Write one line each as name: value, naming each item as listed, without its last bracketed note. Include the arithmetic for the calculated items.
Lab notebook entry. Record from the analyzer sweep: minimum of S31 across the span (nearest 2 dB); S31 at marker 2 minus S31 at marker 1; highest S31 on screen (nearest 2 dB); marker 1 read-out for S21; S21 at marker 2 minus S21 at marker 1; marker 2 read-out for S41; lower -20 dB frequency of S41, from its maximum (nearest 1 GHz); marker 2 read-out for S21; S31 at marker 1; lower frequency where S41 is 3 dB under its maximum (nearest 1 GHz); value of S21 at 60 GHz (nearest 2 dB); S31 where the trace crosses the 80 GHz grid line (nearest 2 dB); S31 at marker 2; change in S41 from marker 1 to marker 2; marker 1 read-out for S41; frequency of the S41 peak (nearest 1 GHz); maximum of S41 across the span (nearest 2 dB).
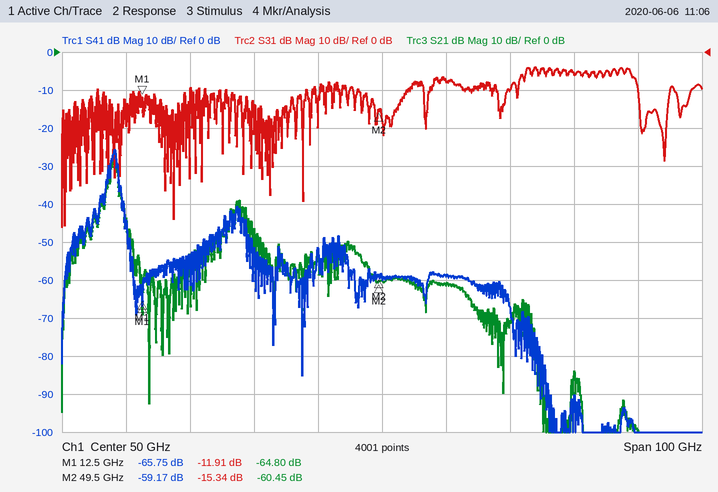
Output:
minimum of S31 across the span: -46 dB
S31 at marker 2 minus S31 at marker 1: -15.34 − (-11.91) = -3.43 dB
highest S31 on screen: -4 dB
marker 1 read-out for S21: -64.80 dB
S21 at marker 2 minus S21 at marker 1: -60.45 − (-64.8) = 4.35 dB
marker 2 read-out for S41: -59.17 dB
lower -20 dB frequency of S41, from its maximum: 5 GHz
marker 2 read-out for S21: -60.45 dB
S31 at marker 1: -11.91 dB
lower frequency where S41 is 3 dB under its maximum: 8 GHz
value of S21 at 60 GHz: -62 dB
S31 where the trace crosses the 80 GHz grid line: -6 dB
S31 at marker 2: -15.34 dB
change in S41 from marker 1 to marker 2: -59.17 − (-65.75) = 6.58 dB
marker 1 read-out for S41: -65.75 dB
frequency of the S41 peak: 8 GHz
maximum of S41 across the span: -26 dB
